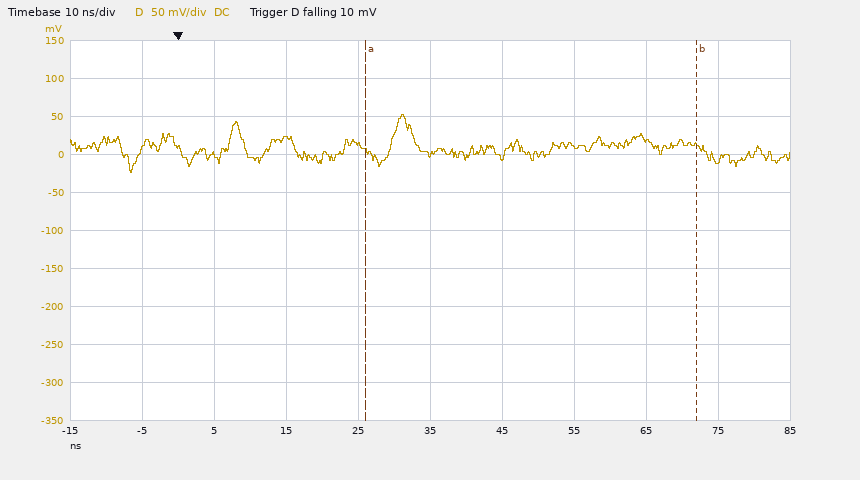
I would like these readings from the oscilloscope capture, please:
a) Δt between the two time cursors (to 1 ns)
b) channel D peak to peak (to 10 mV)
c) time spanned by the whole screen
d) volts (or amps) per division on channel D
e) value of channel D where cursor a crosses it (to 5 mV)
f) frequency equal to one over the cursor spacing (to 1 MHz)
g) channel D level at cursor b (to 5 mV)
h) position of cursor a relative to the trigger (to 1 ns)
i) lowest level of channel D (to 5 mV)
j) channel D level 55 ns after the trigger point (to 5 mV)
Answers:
46 ns
80 mV
100 ns
50 mV
5 mV
22 MHz
10 mV
+26 ns
-25 mV
10 mV
